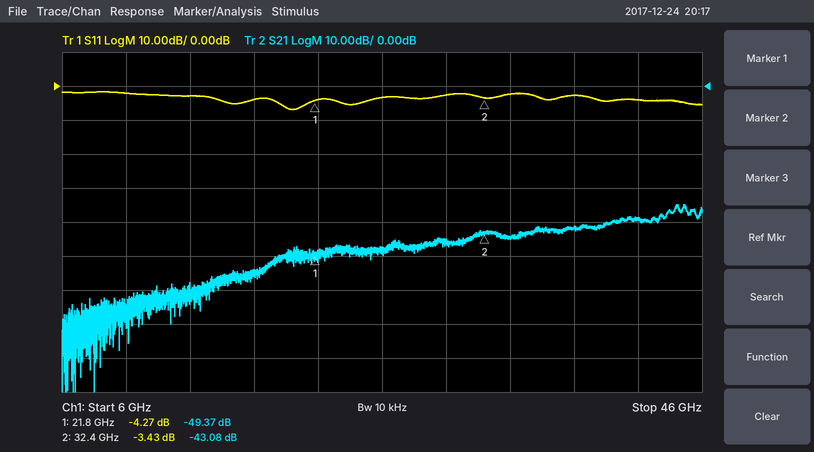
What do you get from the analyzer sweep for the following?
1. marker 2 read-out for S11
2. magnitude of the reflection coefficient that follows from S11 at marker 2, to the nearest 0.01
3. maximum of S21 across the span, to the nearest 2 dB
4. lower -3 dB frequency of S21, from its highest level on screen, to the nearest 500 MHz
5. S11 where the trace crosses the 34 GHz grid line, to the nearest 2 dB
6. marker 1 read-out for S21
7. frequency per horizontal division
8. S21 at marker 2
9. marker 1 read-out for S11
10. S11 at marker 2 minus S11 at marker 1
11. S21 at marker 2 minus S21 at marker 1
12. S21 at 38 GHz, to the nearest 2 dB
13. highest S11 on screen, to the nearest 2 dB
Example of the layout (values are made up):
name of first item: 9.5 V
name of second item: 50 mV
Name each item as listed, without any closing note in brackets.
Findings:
marker 2 read-out for S11: -3.43 dB
magnitude of the reflection coefficient that follows from S11 at marker 2, to the nearest 0.01: 0.67
maximum of S21 across the span, to the nearest 2 dB: -34 dB
lower -3 dB frequency of S21, from its highest level on screen, to the nearest 500 MHz: 44.0 GHz
S11 where the trace crosses the 34 GHz grid line, to the nearest 2 dB: -2 dB
marker 1 read-out for S21: -49.37 dB
frequency per horizontal division: 4 GHz
S21 at marker 2: -43.08 dB
marker 1 read-out for S11: -4.27 dB
S11 at marker 2 minus S11 at marker 1: 0.84 dB
S21 at marker 2 minus S21 at marker 1: 6.29 dB
S21 at 38 GHz, to the nearest 2 dB: -42 dB
highest S11 on screen, to the nearest 2 dB: -2 dB
